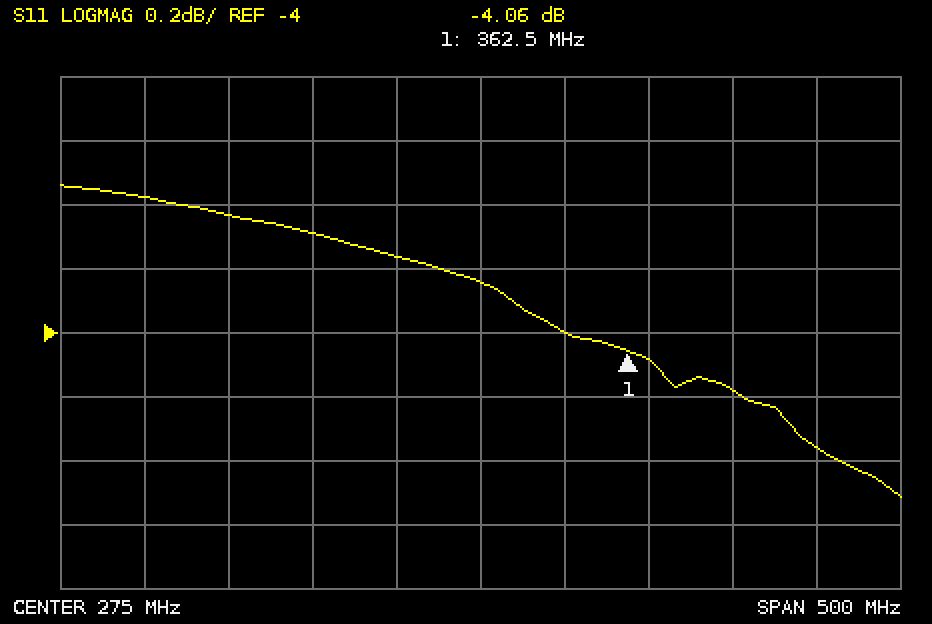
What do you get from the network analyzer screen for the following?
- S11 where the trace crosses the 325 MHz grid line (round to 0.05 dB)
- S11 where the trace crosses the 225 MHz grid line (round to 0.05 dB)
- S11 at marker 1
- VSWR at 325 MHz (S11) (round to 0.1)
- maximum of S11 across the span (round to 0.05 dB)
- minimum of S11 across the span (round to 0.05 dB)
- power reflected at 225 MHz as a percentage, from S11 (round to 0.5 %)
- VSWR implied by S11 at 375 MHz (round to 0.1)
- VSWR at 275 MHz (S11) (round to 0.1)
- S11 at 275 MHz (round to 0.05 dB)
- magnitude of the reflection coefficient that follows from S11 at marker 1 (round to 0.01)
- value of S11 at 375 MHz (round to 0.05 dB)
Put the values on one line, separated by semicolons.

-4.00 dB; -3.75 dB; -4.06 dB; 4.4; -3.55 dB; -4.50 dB; 42.0 %; 4.3; 4.6; -3.85 dB; 0.63; -4.10 dB
